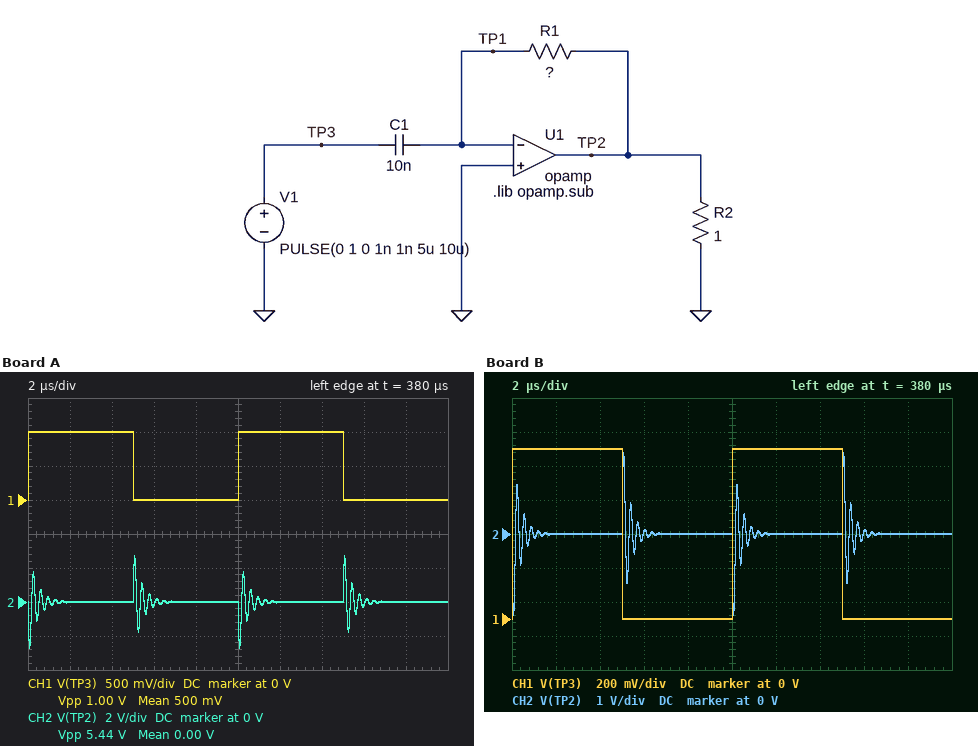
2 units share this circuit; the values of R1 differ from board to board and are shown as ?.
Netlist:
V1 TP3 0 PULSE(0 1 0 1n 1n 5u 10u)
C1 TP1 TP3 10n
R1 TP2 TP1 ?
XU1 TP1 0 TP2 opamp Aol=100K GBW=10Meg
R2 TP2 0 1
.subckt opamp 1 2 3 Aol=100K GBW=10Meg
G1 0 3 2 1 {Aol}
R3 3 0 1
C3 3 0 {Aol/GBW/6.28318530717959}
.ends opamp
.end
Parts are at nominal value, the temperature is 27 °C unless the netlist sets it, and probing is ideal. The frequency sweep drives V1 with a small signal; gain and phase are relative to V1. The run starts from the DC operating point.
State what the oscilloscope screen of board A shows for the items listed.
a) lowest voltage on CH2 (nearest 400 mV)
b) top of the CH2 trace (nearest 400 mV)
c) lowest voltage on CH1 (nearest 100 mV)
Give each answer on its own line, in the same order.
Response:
-2.8 V
2.8 V
0 V
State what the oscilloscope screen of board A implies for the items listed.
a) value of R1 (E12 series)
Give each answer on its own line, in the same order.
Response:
18 Ω
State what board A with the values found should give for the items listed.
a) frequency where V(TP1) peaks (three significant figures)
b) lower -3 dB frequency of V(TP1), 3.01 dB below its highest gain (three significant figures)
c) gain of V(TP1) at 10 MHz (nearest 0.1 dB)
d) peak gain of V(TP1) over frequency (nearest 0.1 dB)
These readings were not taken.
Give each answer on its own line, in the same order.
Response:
3.04 MHz
2.66 MHz
0.8 dB
10.6 dB
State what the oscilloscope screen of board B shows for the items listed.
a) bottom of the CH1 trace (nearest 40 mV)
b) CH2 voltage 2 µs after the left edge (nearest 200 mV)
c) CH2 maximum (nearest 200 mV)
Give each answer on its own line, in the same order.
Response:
0 V
0 V
2.4 V
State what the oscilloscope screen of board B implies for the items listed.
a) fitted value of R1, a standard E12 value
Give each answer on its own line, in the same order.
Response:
15 Ω
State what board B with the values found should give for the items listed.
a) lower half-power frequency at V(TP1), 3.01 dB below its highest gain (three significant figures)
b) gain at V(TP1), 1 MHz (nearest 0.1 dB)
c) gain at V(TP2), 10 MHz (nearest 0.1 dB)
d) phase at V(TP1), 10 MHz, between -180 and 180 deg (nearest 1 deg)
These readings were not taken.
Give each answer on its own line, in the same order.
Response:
2.89 MHz
-19.7 dB
0.9 dB
7 deg
